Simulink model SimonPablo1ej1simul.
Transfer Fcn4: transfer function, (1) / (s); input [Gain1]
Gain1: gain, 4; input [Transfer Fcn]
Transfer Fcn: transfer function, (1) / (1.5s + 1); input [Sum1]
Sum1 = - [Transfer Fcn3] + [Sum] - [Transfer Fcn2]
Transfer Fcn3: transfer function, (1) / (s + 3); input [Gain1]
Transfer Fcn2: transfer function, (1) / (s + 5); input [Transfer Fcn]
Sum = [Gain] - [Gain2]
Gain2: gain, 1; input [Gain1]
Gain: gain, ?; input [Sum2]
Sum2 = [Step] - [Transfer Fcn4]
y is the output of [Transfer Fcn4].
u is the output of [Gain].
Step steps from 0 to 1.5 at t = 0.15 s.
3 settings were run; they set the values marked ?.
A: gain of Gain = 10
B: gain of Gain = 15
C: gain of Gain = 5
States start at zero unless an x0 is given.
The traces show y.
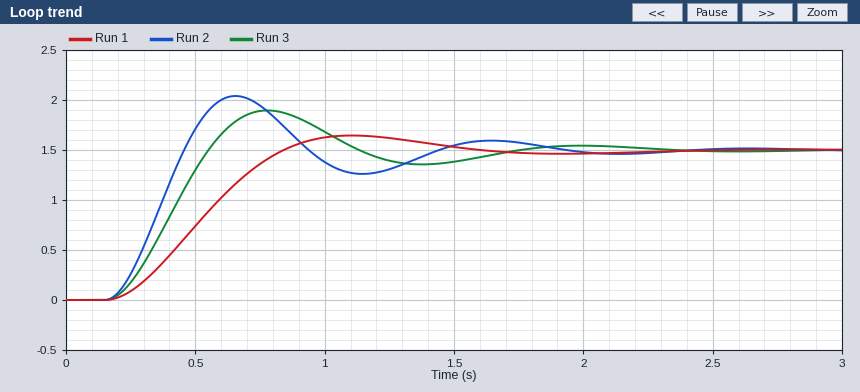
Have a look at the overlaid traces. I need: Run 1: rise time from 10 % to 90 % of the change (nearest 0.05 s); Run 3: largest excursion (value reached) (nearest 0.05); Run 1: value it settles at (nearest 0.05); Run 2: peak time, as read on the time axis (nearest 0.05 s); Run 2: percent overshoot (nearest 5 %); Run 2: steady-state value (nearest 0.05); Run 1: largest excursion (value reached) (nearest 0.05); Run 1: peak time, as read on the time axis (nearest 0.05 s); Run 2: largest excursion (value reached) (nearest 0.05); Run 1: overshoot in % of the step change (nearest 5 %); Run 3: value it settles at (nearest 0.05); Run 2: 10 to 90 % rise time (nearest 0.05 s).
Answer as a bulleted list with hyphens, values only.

- 0.45 s
- 1.90
- 1.50
- 0.65 s
- 35 %
- 1.50
- 1.65
- 1.10 s
- 2.05
- 10 %
- 1.50
- 0.20 s
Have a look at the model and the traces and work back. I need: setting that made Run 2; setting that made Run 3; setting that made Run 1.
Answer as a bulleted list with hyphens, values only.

- B
- A
- C
